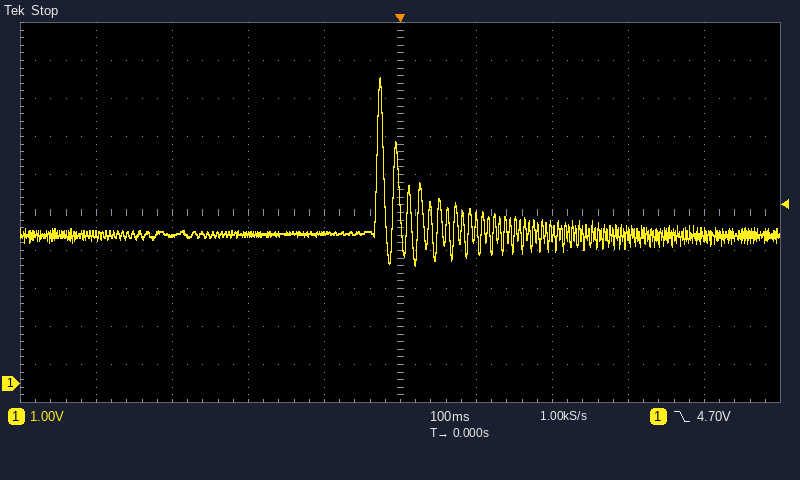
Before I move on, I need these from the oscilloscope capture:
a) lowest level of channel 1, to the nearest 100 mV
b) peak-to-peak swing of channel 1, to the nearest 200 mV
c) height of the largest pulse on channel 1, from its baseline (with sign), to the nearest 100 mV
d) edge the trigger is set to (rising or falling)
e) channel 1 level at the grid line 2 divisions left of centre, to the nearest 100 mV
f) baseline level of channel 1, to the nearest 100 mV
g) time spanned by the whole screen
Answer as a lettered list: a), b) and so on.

a) 3.1 V
b) 5.0 V
c) +4.1 V
d) falling
e) 3.9 V
f) 3.9 V
g) 1 s
